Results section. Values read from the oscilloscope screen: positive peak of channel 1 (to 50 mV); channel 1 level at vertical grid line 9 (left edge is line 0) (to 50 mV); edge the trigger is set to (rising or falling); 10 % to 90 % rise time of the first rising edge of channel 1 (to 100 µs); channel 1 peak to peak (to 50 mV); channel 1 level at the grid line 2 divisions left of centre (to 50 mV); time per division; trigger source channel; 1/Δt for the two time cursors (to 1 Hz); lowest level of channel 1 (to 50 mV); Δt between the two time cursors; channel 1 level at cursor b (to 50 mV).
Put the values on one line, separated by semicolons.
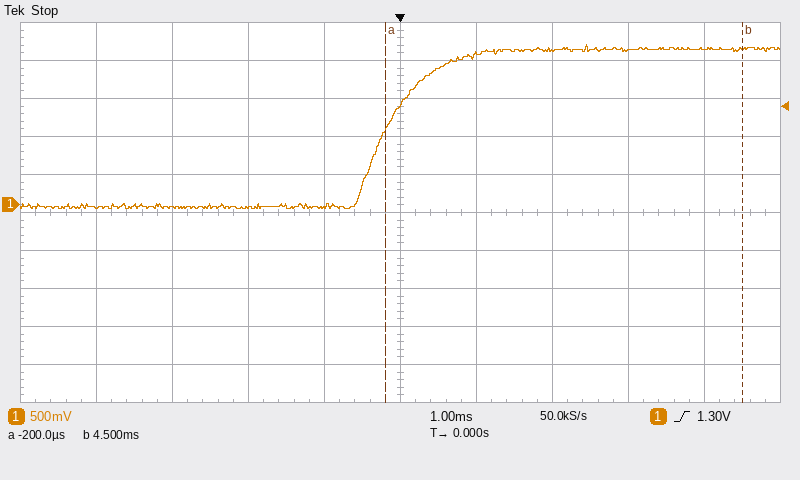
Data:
2.10 V; 2.05 V; rising; 1.1 ms; 2.15 V; -50 mV; 1 ms; channel 1; 213 Hz; -50 mV; 4.7 ms; 2.05 V
